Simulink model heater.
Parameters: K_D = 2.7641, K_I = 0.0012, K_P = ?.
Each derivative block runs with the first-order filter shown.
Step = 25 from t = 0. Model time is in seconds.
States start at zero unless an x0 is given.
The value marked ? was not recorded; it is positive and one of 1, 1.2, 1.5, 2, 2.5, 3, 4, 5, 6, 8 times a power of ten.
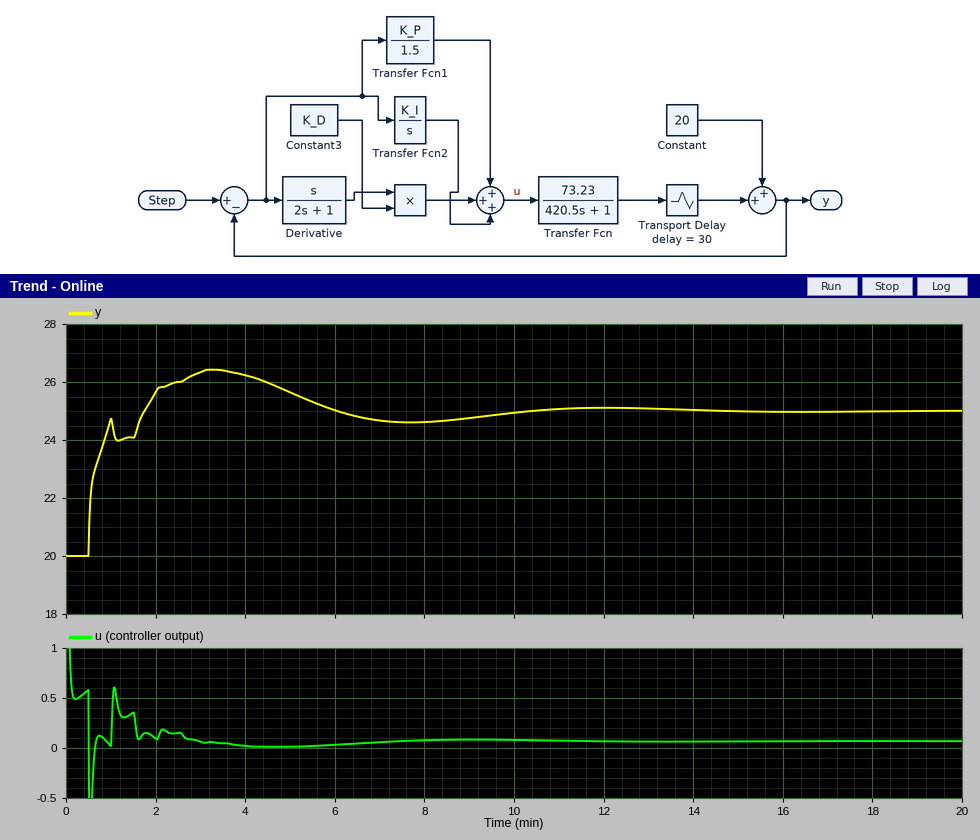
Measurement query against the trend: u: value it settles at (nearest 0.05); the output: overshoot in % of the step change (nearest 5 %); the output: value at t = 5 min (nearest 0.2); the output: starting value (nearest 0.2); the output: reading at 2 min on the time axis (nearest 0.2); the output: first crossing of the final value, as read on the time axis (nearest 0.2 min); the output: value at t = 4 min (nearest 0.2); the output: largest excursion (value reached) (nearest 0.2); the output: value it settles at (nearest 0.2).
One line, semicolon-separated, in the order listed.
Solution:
0.05; 30 %; 25.6; 20.0; 25.6; 1.8 min; 26.2; 26.4; 25.0
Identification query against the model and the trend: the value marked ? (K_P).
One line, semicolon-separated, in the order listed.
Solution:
0.12
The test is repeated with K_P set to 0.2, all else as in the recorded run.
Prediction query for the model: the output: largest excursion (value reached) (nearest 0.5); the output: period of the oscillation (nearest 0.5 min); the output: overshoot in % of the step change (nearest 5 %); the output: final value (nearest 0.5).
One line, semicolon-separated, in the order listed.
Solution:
26.0; 1.5 min; 20 %; 25.0
